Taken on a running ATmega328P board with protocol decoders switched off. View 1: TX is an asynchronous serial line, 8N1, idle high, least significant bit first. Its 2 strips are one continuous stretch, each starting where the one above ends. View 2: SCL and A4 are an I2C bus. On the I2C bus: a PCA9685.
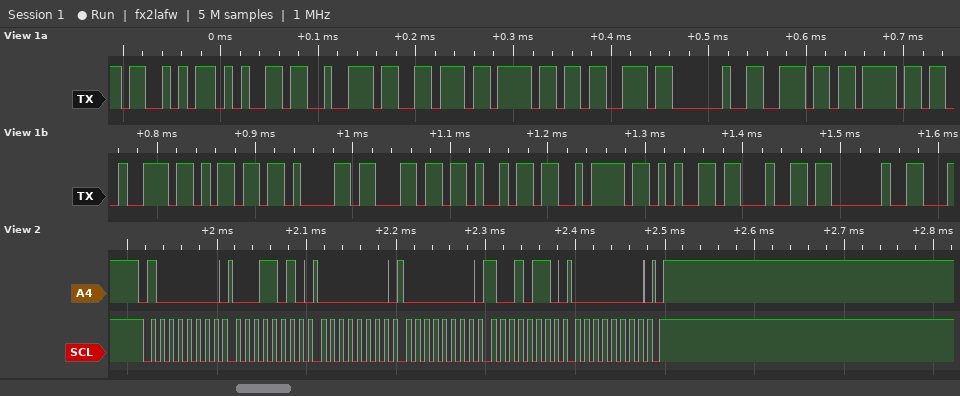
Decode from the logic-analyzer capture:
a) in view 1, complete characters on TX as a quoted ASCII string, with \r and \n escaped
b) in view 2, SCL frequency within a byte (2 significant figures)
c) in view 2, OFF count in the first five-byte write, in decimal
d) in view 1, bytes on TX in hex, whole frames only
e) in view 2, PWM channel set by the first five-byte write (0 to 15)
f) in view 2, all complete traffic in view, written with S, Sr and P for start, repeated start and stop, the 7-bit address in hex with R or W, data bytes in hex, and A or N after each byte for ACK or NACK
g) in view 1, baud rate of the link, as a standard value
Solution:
"Servos normalized "
100 kHz
150
0x53 0x65 0x72 0x76 0x6F 0x73 0x20 0x6E 0x6F 0x72 0x6D 0x61 0x6C 0x69 0x7A 0x65 0x64 0x20
5
S 40W A 1A A 00 A 00 A 96 A 00 A P
115200 baud
